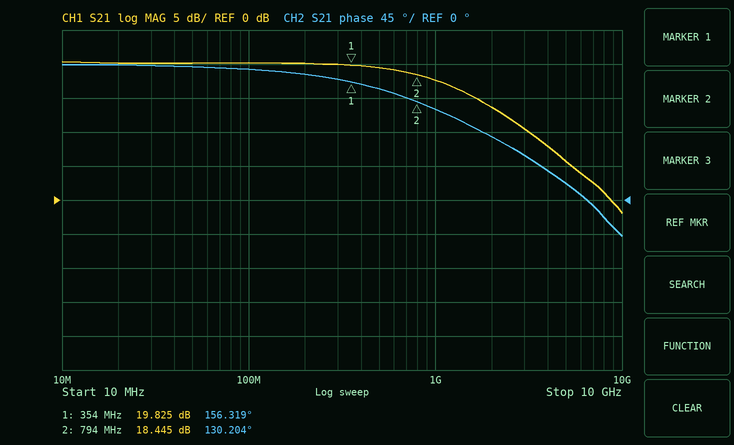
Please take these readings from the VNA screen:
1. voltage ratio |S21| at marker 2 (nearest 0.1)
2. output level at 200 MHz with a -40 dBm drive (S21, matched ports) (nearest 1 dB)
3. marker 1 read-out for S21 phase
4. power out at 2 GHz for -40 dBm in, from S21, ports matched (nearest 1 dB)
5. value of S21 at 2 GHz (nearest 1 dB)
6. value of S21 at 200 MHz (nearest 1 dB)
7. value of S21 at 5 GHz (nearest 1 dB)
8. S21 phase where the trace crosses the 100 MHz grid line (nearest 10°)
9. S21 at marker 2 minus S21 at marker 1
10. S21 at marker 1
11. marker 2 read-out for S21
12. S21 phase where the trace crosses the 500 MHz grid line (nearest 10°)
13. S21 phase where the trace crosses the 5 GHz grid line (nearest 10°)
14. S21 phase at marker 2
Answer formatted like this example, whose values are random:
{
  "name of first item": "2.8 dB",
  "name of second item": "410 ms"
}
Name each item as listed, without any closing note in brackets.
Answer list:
{
  "voltage ratio |S21| at marker 2": "8.4",
  "output level at 200 MHz with a -40 dBm drive (S21, matched ports)": "-20 dBm",
  "marker 1 read-out for S21 phase": "156.319°",
  "power out at 2 GHz for -40 dBm in, from S21, ports matched": "-26 dBm",
  "value of S21 at 2 GHz": "14 dB",
  "value of S21 at 200 MHz": "20 dB",
  "value of S21 at 5 GHz": "6 dB",
  "S21 phase where the trace crosses the 100 MHz grid line": "170°",
  "S21 at marker 2 minus S21 at marker 1": "-1.380 dB",
  "S21 at marker 1": "19.825 dB",
  "marker 2 read-out for S21": "18.445 dB",
  "S21 phase where the trace crosses the 500 MHz grid line": "150°",
  "S21 phase where the trace crosses the 5 GHz grid line": "20°",
  "S21 phase at marker 2": "130.204°"
}
